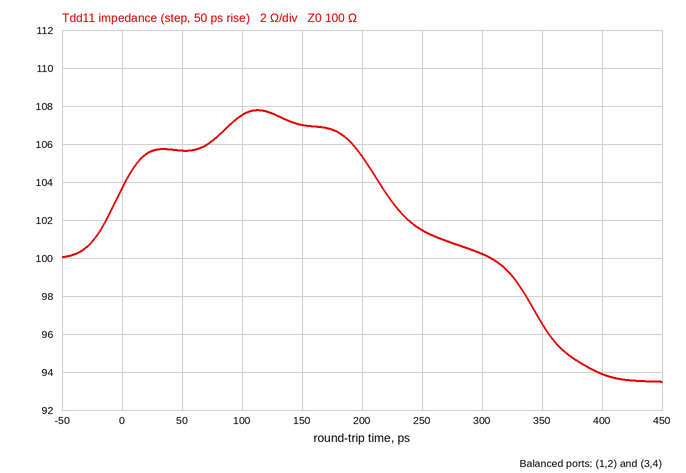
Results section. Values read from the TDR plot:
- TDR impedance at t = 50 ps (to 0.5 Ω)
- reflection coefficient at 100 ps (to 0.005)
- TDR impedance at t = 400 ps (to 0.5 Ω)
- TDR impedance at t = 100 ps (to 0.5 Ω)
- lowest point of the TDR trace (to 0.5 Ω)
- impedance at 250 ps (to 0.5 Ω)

105.5 Ω
+0.035
94.0 Ω
107.5 Ω
93.5 Ω
101.5 Ω
